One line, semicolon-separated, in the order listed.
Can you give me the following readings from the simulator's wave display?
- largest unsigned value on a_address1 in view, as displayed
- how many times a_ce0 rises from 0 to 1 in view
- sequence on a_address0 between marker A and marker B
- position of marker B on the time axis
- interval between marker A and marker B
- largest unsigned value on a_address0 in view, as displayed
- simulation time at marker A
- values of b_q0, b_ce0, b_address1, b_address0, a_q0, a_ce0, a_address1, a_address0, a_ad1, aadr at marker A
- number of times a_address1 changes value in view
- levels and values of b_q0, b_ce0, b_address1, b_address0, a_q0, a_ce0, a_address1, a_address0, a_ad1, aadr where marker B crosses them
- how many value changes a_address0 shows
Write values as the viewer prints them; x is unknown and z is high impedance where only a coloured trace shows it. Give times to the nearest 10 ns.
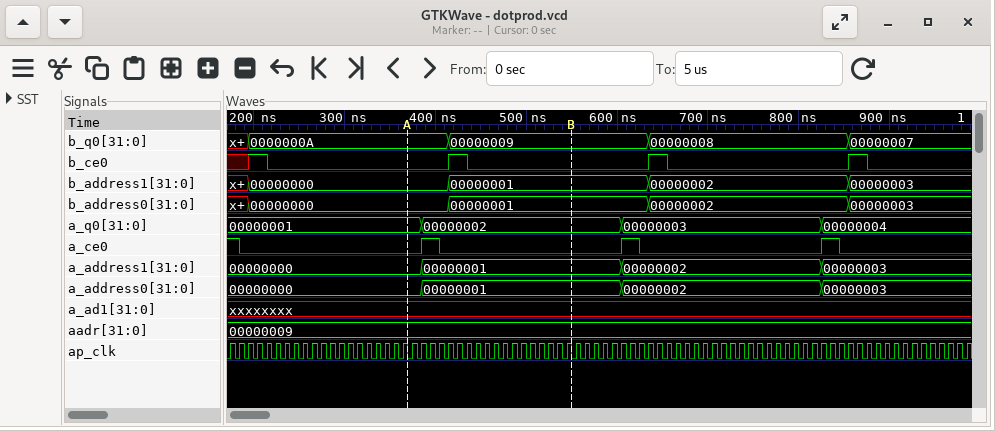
00000003; 3; 00000000, 00000001; 550 ns; 180 ns; 00000003; 370 ns; b_q0=0000000A, b_ce0=0, b_address1=00000000, b_address0=00000000, a_q0=00000001, a_ce0=0, a_address1=00000000, a_address0=00000000, a_ad1=xxxxxxxx, aadr=00000009; 3; b_q0=00000009, b_ce0=0, b_address1=00000001, b_address0=00000001, a_q0=00000002, a_ce0=0, a_address1=00000001, a_address0=00000001, a_ad1=xxxxxxxx, aadr=00000009; 3
